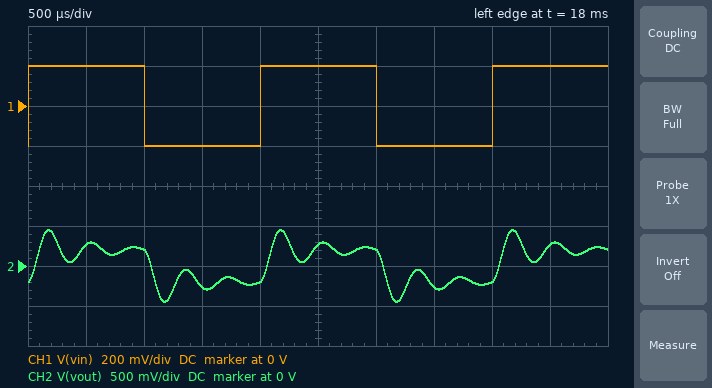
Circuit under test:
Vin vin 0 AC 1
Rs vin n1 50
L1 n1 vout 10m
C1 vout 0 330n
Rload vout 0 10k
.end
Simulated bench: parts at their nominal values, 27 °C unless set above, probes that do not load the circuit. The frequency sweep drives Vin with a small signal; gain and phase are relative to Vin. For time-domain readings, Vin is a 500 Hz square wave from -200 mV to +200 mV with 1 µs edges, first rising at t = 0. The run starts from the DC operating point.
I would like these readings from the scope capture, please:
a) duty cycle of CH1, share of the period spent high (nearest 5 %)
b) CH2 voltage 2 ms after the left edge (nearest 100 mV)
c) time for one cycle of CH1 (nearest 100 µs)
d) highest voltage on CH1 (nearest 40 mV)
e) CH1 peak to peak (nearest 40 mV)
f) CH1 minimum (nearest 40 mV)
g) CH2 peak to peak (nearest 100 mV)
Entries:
50 %
-200 mV
2.0 ms
200 mV
400 mV
-200 mV
900 mV
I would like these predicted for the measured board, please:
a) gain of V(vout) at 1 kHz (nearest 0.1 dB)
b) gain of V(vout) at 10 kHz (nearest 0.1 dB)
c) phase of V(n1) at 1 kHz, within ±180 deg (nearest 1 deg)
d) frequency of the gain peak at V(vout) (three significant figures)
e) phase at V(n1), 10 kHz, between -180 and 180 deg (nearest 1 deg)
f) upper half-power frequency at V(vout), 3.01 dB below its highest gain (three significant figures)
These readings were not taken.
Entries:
1.1 dB
-21.6 dB
-7 deg
2.71 kHz
5 deg
3.11 kHz
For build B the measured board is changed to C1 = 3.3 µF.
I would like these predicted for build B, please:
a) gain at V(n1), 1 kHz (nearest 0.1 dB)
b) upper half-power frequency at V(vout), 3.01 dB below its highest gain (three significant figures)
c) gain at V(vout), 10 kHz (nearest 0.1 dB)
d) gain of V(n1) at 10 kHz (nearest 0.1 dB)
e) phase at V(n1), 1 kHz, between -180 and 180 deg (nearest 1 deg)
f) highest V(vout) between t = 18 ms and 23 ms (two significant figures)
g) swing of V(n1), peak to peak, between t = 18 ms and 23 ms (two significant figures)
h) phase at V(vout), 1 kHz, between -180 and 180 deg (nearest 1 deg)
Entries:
-11.1 dB
1.04 kHz
-42.3 dB
0 dB
73 deg
280 mV
480 mV
-106 deg
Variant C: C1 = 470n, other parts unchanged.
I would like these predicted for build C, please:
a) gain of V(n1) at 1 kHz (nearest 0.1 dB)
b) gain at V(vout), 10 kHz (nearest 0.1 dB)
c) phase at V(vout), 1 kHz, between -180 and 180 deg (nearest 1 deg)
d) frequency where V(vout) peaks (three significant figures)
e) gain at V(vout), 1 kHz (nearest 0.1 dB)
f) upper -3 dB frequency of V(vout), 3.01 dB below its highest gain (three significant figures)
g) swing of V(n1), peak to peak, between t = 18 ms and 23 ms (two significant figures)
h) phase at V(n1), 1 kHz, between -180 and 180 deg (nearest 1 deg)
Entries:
-0.2 dB
-24.9 dB
-11 deg
2.25 kHz
1.6 dB
2.64 kHz
520 mV
-10 deg
